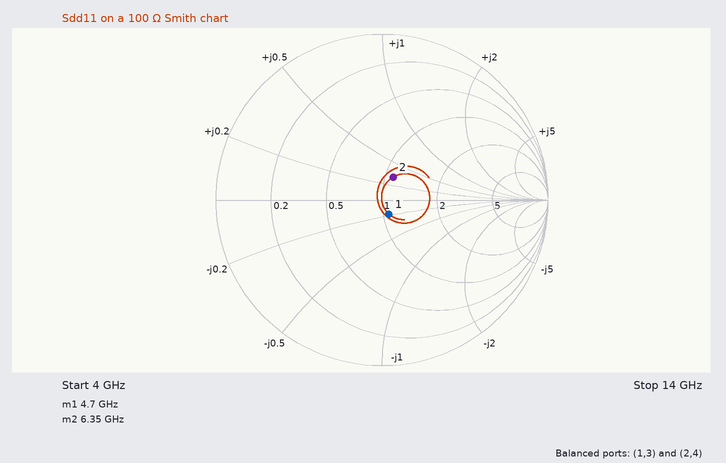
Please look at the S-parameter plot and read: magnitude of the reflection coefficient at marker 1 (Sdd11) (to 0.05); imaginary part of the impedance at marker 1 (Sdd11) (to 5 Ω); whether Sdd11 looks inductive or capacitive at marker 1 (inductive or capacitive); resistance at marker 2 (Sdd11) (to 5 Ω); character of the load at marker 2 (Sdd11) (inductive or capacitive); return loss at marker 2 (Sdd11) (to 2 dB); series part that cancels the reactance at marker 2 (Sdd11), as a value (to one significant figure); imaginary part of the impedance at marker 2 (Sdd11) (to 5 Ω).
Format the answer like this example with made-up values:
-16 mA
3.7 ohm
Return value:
0.10
-20 Ω
capacitive
110 Ω
inductive
16 dB
800 fF
+30 Ω
